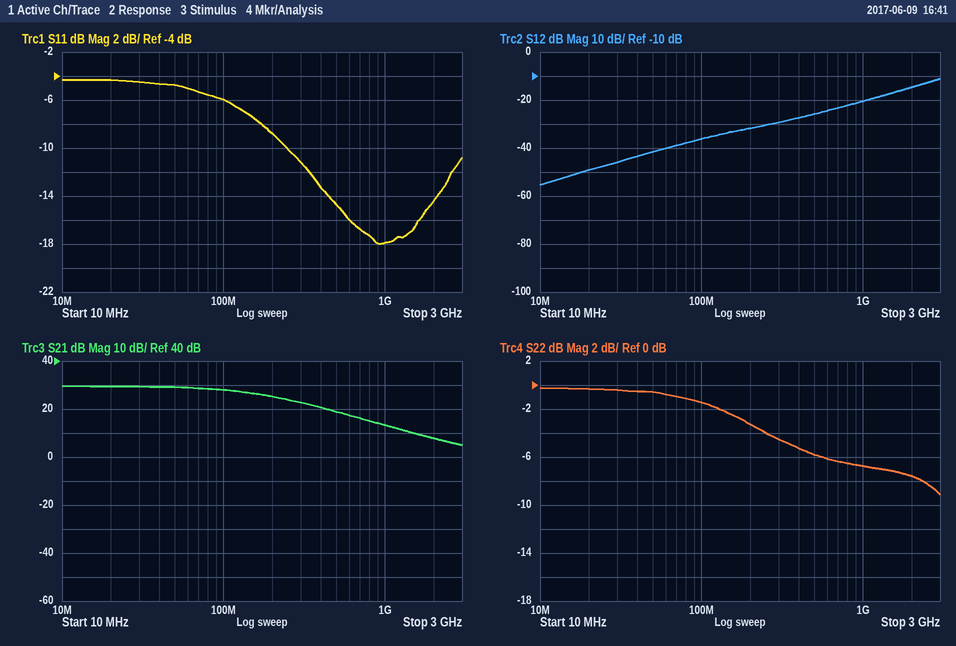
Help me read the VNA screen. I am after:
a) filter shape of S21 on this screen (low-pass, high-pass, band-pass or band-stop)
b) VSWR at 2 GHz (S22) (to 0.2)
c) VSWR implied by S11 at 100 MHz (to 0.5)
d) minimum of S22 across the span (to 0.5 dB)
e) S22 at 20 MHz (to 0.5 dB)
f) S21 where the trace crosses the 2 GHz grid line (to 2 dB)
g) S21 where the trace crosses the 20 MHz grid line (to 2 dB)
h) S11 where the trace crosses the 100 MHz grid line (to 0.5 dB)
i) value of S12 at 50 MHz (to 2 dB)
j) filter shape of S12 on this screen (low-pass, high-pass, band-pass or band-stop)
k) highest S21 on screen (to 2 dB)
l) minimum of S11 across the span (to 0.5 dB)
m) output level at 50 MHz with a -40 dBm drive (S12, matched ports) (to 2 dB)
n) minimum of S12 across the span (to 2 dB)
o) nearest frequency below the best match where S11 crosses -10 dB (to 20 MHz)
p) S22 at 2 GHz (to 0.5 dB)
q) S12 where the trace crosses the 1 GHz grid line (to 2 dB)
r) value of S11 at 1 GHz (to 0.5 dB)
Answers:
low-pass
2.4
3.0
-9.0 dB
-0.5 dB
8 dB
30 dB
-6.0 dB
-42 dB
high-pass
30 dB
-18.0 dB
-82 dBm
-56 dB
240 MHz
-7.5 dB
-20 dB
-18.0 dB
